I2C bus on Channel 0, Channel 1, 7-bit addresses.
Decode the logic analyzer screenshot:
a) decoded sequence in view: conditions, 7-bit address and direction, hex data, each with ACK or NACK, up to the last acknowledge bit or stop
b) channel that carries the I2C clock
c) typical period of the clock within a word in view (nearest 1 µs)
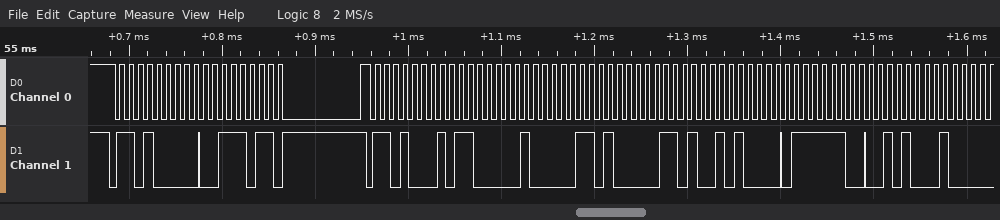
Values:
start, address 68 write ACK, 3B ACK, repeated start, address 68 read ACK, C1 ACK, 0D ACK, 0D ACK, 50 ACK, FC ACK, 51 ACK
Channel 0
10 µs
